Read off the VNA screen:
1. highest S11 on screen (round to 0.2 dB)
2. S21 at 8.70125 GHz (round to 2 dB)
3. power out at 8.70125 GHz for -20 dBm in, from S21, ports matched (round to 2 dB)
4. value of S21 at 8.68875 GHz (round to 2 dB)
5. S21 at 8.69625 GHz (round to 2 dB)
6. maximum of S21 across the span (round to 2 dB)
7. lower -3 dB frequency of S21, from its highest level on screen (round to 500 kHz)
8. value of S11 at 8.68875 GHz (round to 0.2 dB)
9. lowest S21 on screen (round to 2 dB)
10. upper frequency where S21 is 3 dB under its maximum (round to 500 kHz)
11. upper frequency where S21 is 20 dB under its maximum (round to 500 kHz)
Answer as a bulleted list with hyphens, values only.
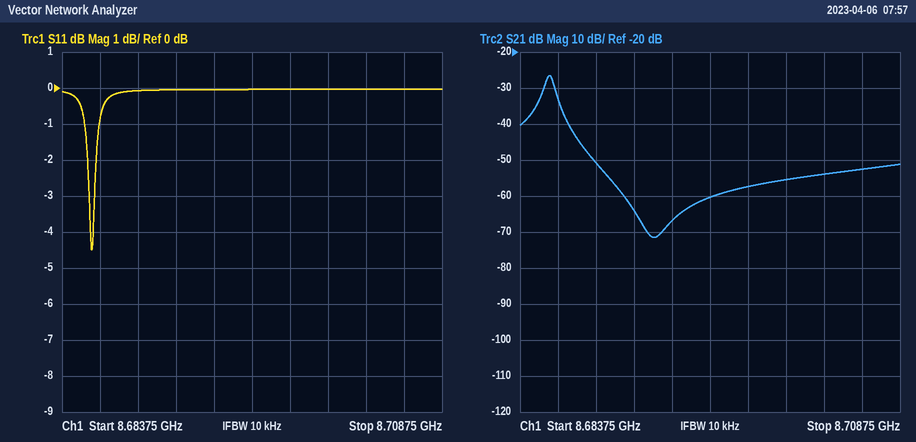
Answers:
- 0.0 dB
- -56 dB
- -76 dBm
- -50 dB
- -60 dB
- -26 dB
- 8.6855 GHz
- 0.0 dB
- -72 dB
- 8.6860 GHz
- 8.6880 GHz
